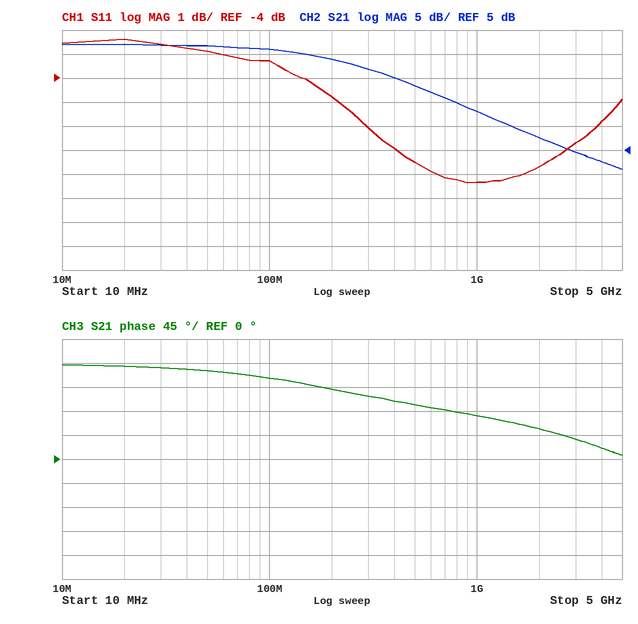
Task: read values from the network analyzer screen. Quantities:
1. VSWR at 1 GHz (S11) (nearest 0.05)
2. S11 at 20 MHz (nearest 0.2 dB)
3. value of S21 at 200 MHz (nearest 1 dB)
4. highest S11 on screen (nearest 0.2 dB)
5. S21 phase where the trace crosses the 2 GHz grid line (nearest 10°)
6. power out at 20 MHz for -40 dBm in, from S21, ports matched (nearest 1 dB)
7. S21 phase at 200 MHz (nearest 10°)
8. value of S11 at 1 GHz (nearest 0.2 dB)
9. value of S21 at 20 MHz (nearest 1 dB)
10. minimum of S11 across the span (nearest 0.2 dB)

2.25
-2.4 dB
24 dB
-2.4 dB
60°
-13 dBm
130°
-8.4 dB
27 dB
-8.4 dB
